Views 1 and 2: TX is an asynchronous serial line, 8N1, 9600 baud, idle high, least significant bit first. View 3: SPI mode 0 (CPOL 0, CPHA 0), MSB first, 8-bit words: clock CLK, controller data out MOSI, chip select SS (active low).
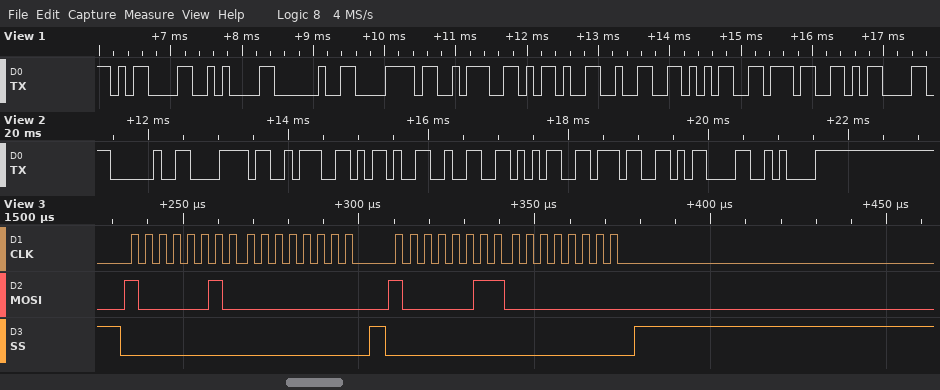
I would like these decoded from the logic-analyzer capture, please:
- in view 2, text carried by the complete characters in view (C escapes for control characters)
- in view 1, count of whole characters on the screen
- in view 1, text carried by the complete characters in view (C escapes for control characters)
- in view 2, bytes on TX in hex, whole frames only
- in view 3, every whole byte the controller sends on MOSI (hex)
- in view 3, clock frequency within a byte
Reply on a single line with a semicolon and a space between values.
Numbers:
" x:-257\r\n"; 10; "\r\n x:-257\r"; 20 78 3A 2D 32 35 37 0D 0A; 82 00 83 00; 250 kHz
